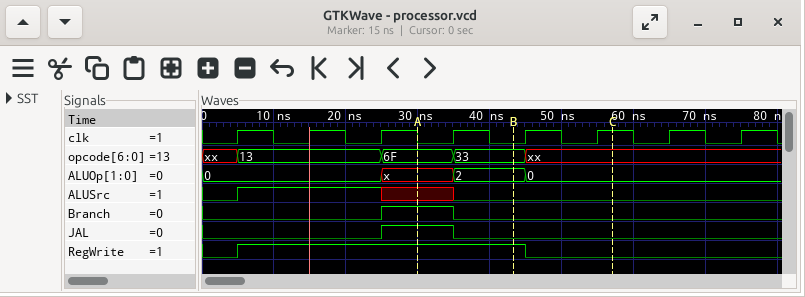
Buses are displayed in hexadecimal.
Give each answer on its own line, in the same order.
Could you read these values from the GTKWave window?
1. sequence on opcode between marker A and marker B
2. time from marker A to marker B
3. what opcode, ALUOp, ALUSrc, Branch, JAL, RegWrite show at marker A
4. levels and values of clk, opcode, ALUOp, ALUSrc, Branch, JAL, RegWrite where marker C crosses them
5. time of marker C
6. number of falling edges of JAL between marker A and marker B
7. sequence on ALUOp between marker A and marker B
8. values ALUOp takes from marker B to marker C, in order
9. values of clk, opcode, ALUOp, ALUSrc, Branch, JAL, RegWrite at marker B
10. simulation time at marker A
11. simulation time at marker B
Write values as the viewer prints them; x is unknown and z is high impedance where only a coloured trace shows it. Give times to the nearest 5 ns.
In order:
6F, 33
15 ns
opcode=6F, ALUOp=x, ALUSrc=x, Branch=1, JAL=1, RegWrite=1
clk=1, opcode=xx, ALUOp=0, ALUSrc=0, Branch=0, JAL=0, RegWrite=0
55 ns
1
x, 2
2, 0
clk=0, opcode=33, ALUOp=2, ALUSrc=0, Branch=0, JAL=0, RegWrite=1
30 ns
45 ns
